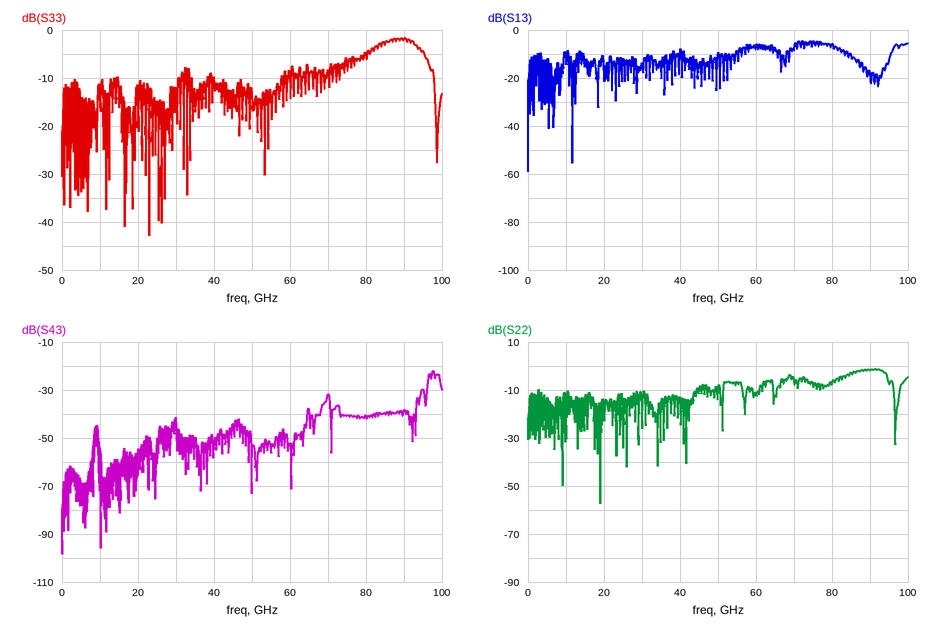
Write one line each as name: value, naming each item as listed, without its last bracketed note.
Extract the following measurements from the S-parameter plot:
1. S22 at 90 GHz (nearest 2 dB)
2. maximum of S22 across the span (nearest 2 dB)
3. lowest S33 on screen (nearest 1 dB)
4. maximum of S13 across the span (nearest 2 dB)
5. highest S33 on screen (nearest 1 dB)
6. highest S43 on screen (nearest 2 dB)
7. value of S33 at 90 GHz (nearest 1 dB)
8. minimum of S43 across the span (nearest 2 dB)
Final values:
S22 at 90 GHz: -2 dB
maximum of S22 across the span: -2 dB
lowest S33 on screen: -43 dB
maximum of S13 across the span: -4 dB
highest S33 on screen: -2 dB
highest S43 on screen: -22 dB
value of S33 at 90 GHz: -2 dB
minimum of S43 across the span: -98 dB
